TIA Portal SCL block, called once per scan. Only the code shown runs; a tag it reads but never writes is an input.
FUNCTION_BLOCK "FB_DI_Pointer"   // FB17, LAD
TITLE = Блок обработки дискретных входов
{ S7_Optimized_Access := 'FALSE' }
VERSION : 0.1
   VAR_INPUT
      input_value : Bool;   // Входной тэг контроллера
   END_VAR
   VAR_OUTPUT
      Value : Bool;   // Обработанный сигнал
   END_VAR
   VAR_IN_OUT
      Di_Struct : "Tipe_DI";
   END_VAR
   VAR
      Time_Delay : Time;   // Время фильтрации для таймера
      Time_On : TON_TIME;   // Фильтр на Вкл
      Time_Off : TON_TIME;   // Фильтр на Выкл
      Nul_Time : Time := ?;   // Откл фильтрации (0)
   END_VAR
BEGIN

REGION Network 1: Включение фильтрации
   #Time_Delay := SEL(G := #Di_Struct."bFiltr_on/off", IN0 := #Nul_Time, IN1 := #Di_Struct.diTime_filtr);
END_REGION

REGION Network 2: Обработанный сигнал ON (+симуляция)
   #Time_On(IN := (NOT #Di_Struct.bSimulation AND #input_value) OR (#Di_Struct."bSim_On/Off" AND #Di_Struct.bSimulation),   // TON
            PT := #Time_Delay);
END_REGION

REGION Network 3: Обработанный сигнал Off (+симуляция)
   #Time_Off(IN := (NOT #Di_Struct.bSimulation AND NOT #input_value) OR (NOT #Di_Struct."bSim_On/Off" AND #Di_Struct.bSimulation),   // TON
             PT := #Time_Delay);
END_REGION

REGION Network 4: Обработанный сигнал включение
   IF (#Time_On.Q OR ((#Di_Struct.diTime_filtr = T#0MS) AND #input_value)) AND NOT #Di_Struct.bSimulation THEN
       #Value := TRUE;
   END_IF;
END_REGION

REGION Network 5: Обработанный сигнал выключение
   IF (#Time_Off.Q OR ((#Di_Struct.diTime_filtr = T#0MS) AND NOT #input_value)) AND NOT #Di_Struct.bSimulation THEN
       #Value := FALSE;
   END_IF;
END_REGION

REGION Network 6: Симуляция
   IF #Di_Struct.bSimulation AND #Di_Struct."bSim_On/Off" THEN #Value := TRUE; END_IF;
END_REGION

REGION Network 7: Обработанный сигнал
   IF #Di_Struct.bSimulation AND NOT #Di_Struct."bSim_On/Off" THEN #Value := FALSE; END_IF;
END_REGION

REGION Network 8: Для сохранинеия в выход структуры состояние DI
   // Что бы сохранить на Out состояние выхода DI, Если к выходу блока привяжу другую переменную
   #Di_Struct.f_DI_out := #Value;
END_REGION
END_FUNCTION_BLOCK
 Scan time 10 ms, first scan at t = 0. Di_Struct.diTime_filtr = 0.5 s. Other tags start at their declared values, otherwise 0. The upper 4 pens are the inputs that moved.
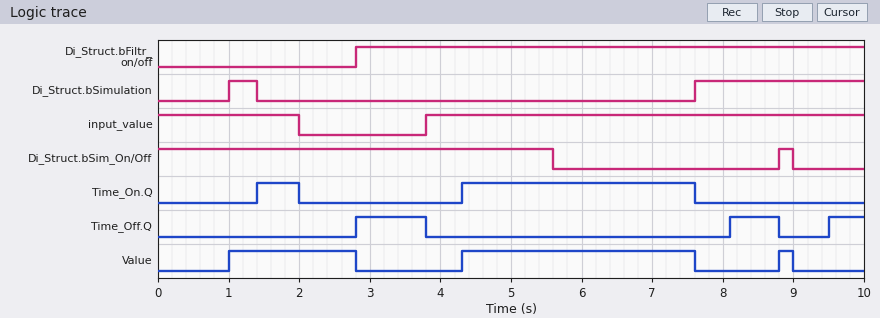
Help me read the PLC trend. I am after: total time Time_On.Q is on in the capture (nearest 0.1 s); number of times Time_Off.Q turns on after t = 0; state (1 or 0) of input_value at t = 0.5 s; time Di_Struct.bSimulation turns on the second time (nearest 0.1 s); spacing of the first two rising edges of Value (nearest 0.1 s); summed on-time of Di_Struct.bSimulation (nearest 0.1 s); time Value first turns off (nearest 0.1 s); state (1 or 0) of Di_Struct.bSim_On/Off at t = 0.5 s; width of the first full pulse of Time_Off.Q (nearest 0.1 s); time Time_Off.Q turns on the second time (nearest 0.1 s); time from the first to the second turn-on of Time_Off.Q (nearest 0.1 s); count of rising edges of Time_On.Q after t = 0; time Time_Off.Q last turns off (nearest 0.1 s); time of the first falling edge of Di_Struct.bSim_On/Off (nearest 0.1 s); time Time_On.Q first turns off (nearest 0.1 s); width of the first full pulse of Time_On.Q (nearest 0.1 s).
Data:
3.9 s
3
1
7.6 s
3.3 s
2.8 s
2.8 s
1
1.0 s
8.1 s
5.3 s
2
8.8 s
5.6 s
2.0 s
0.6 s
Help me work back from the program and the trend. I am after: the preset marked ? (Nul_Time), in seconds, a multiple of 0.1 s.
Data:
1.4 s
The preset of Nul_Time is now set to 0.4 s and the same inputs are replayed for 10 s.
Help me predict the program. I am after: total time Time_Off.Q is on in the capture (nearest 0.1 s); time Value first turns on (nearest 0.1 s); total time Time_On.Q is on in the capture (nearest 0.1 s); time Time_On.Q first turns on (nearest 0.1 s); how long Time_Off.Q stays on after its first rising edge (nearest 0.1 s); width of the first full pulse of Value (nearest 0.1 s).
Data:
2.6 s
0.4 s
4.9 s
0.4 s
1.4 s
2.0 s
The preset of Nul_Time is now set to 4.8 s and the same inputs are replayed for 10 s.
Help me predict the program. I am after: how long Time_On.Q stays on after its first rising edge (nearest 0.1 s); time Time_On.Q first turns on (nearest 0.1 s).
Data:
3.3 s
4.3 s
